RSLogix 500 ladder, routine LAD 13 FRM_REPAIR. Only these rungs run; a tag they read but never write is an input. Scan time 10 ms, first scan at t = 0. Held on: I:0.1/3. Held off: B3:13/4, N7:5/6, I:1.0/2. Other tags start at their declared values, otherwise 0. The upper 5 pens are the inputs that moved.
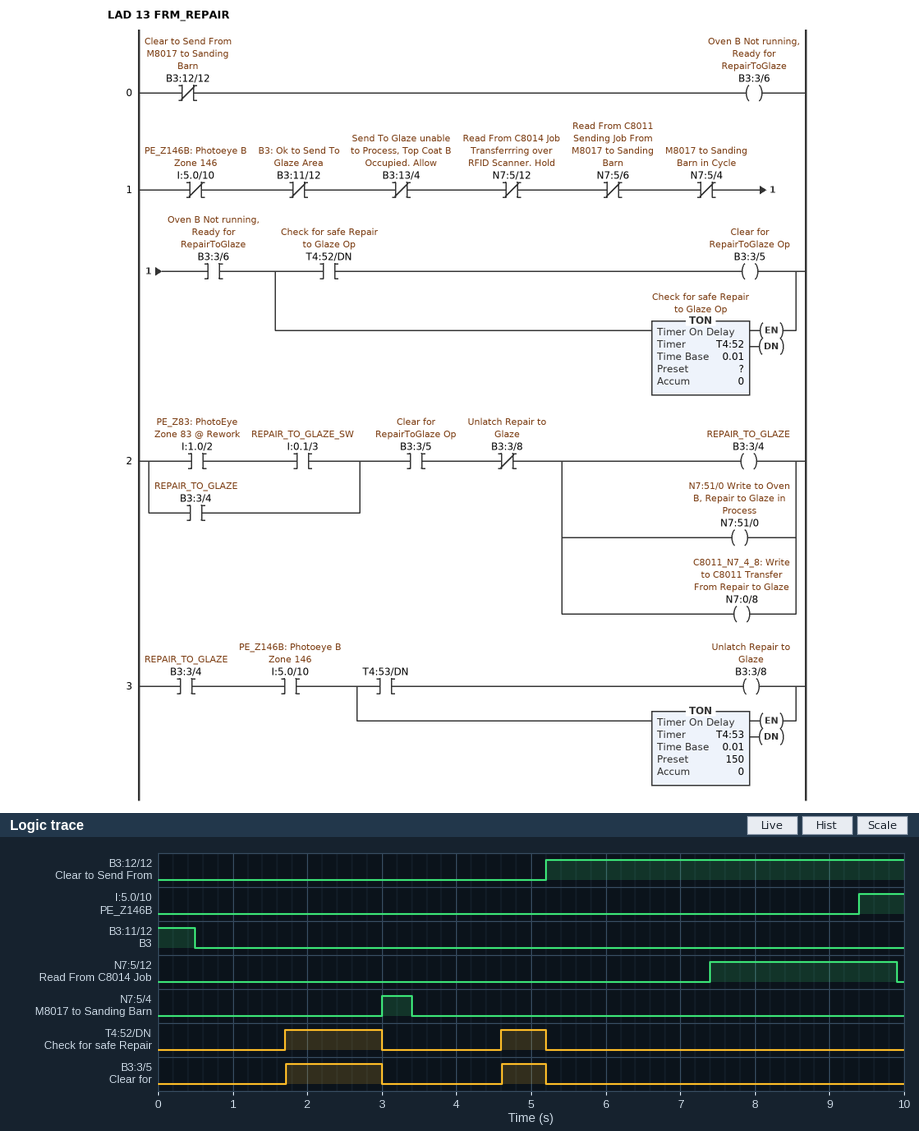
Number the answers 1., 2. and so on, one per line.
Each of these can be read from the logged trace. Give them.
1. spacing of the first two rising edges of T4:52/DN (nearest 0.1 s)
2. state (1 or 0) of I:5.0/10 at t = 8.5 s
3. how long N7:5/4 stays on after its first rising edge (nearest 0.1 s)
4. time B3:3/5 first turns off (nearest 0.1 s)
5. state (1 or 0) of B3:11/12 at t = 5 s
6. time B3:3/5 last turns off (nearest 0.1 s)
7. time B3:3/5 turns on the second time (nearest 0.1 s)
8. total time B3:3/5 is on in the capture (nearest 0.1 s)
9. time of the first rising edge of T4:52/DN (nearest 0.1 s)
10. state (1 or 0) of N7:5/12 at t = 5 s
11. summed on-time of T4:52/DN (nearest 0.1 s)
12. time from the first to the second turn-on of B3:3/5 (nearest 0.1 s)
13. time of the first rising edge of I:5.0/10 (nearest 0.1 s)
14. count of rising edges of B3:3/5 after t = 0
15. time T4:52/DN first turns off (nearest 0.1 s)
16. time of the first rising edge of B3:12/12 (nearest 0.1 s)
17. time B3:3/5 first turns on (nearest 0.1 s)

1. 2.9 s
2. 0
3. 0.4 s
4. 3.0 s
5. 0
6. 5.2 s
7. 4.6 s
8. 1.9 s
9. 1.7 s
10. 0
11. 1.9 s
12. 2.9 s
13. 9.4 s
14. 2
15. 3.0 s
16. 5.2 s
17. 1.7 s
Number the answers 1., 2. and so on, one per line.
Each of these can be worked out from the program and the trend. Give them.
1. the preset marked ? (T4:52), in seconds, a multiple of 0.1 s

1. 1.2 s
